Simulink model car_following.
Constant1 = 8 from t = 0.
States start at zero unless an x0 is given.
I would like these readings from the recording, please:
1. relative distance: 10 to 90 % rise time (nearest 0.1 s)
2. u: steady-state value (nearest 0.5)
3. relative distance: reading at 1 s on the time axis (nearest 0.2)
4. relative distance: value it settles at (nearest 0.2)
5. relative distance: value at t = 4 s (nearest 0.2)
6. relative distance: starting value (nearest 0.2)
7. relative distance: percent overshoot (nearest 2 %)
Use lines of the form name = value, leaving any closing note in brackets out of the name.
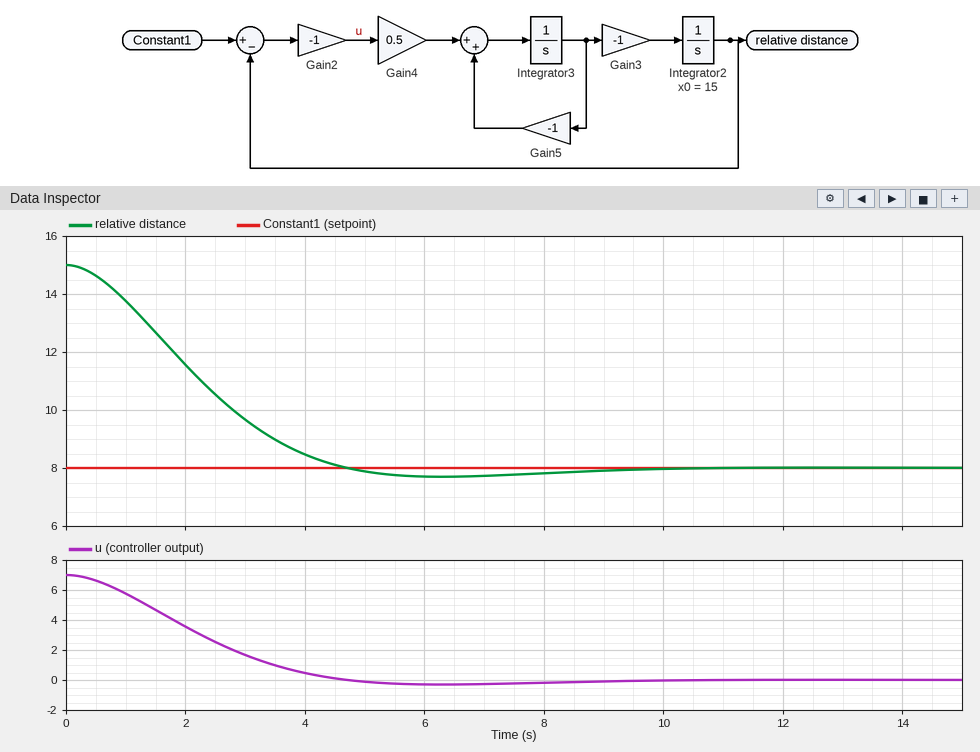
relative distance: 10 to 90 % rise time = 3.0 s
u: steady-state value = 0.0
relative distance: reading at 1 s on the time axis = 13.8
relative distance: value it settles at = 8.0
relative distance: value at t = 4 s = 8.4
relative distance: starting value = 15.0
relative distance: percent overshoot = 4 %
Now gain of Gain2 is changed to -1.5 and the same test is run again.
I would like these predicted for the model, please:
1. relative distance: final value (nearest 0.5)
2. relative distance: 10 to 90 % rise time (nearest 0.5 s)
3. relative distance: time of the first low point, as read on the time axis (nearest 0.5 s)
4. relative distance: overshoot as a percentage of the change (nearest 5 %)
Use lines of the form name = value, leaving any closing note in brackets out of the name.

relative distance: final value = 8.0
relative distance: 10 to 90 % rise time = 2.0 s
relative distance: time of the first low point, as read on the time axis = 4.5 s
relative distance: overshoot as a percentage of the change = 10 %
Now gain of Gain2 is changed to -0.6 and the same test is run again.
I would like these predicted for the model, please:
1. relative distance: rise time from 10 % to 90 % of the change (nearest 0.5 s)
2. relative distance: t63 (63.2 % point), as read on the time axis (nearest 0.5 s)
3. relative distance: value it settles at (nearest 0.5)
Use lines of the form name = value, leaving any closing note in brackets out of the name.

relative distance: rise time from 10 % to 90 % of the change = 5.5 s
relative distance: t63 (63.2 % point), as read on the time axis = 3.5 s
relative distance: value it settles at = 8.0
